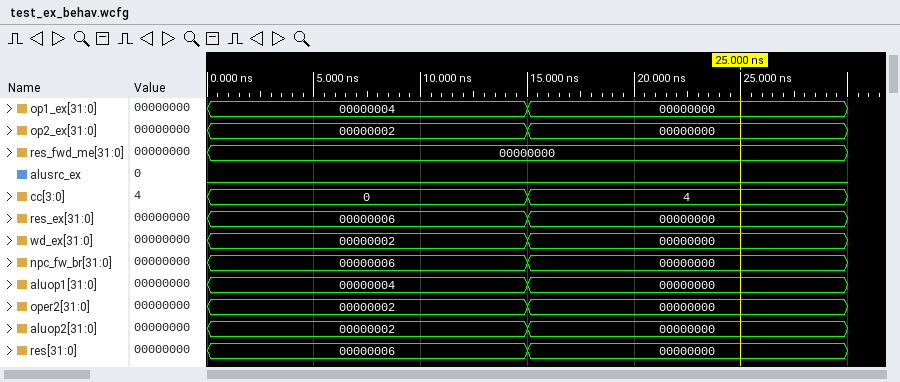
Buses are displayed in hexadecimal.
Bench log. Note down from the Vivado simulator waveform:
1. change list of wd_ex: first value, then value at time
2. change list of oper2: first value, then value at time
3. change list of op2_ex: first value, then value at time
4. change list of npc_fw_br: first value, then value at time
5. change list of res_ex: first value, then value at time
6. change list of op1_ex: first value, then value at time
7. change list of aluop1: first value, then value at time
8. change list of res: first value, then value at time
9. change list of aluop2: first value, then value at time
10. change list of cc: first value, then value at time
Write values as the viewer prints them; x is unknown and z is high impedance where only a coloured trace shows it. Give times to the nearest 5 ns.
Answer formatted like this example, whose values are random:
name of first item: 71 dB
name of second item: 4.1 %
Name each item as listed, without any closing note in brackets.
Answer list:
change list of wd_ex: first value, then value at time: 00000002, 00000000 at 15 ns
change list of oper2: first value, then value at time: 00000002, 00000000 at 15 ns
change list of op2_ex: first value, then value at time: 00000002, 00000000 at 15 ns
change list of npc_fw_br: first value, then value at time: 00000006, 00000000 at 15 ns
change list of res_ex: first value, then value at time: 00000006, 00000000 at 15 ns
change list of op1_ex: first value, then value at time: 00000004, 00000000 at 15 ns
change list of aluop1: first value, then value at time: 00000004, 00000000 at 15 ns
change list of res: first value, then value at time: 00000006, 00000000 at 15 ns
change list of aluop2: first value, then value at time: 00000002, 00000000 at 15 ns
change list of cc: first value, then value at time: 0, 4 at 15 ns
